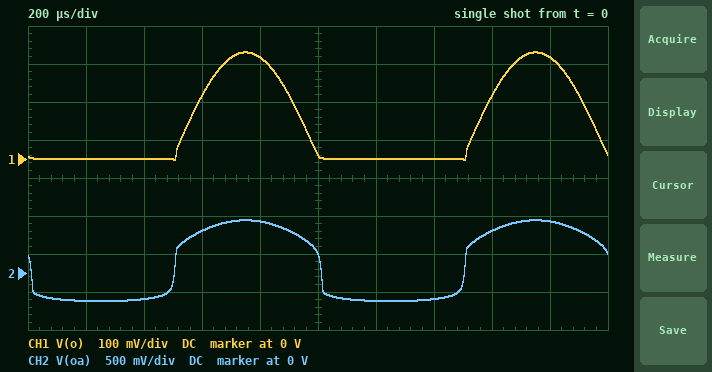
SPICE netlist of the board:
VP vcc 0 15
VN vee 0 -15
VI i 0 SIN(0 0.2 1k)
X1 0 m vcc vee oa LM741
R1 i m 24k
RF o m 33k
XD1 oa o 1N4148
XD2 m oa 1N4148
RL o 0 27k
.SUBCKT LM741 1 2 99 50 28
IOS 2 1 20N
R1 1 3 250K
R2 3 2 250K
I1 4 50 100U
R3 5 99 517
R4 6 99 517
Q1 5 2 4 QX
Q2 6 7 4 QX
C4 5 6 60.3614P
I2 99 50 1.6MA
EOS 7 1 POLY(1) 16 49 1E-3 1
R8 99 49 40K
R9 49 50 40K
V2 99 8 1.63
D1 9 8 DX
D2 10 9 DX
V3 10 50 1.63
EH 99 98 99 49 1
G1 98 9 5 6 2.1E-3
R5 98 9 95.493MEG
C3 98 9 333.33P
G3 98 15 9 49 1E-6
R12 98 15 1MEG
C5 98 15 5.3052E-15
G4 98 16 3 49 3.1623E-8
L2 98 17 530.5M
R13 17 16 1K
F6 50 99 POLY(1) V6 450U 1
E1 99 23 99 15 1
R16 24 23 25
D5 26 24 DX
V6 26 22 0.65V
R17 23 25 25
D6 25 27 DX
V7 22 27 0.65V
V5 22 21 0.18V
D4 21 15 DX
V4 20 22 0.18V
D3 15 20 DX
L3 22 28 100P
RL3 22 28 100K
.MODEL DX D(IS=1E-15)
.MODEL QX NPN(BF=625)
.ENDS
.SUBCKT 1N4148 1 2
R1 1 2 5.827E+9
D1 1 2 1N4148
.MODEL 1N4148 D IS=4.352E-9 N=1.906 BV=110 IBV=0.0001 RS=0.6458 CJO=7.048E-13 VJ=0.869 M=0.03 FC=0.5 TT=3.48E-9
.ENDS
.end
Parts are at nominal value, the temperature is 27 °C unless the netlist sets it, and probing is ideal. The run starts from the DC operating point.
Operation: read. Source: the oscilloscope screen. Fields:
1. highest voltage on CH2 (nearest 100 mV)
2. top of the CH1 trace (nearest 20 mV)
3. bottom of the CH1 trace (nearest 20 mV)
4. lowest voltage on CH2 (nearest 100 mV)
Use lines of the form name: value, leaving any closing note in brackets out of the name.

highest voltage on CH2: 700 mV
top of the CH1 trace: 280 mV
bottom of the CH1 trace: 0 V
lowest voltage on CH2: -400 mV
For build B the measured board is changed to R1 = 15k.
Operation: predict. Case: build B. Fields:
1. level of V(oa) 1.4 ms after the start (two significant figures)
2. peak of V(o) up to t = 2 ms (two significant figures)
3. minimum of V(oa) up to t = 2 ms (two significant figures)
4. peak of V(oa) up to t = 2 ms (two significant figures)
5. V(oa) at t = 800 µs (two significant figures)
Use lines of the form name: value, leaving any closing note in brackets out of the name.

level of V(oa) 1.4 ms after the start: -370 mV
peak of V(o) up to t = 2 ms: 450 mV
minimum of V(oa) up to t = 2 ms: -390 mV
peak of V(oa) up to t = 2 ms: 880 mV
V(oa) at t = 800 µs: 860 mV
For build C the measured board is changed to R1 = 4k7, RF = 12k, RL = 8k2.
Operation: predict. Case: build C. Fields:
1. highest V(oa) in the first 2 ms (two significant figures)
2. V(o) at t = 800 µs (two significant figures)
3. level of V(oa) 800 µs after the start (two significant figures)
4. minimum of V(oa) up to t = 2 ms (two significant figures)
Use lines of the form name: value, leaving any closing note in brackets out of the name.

highest V(oa) in the first 2 ms: 1.0 V
V(o) at t = 800 µs: 490 mV
level of V(oa) 800 µs after the start: 990 mV
minimum of V(oa) up to t = 2 ms: -450 mV
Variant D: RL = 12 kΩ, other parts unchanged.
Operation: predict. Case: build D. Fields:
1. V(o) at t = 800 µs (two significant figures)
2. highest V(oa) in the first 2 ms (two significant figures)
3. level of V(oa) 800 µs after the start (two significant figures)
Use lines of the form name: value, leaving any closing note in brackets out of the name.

V(o) at t = 800 µs: 270 mV
highest V(oa) in the first 2 ms: 720 mV
level of V(oa) 800 µs after the start: 700 mV
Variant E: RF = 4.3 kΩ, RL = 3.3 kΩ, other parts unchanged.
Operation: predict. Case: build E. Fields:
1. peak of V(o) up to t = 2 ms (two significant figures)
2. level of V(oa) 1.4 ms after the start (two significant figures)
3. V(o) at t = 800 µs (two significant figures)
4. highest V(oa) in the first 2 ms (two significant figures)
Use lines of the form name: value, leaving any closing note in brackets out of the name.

peak of V(o) up to t = 2 ms: 37 mV
level of V(oa) 1.4 ms after the start: -340 mV
V(o) at t = 800 µs: 36 mV
highest V(oa) in the first 2 ms: 450 mV
